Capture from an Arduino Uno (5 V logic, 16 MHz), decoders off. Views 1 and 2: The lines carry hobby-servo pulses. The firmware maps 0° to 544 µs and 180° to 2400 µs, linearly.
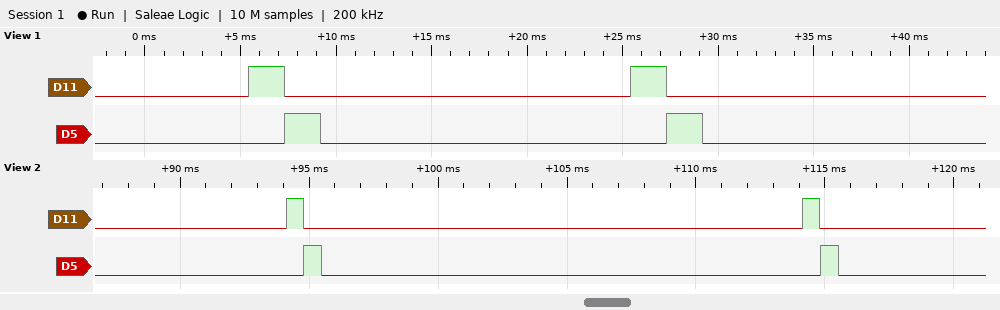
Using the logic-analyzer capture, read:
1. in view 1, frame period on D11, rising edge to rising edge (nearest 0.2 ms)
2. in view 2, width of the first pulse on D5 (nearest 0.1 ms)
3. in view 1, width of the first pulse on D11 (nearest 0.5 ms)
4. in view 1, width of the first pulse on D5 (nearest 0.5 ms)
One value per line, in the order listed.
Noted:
20.0 ms
0.7 ms
2.0 ms
2.0 ms
